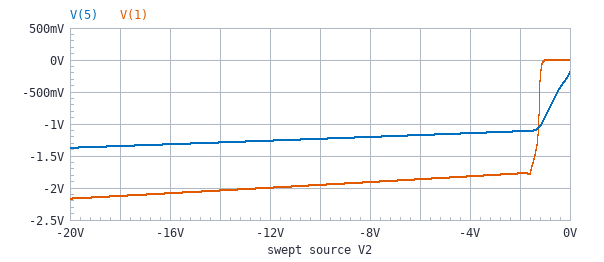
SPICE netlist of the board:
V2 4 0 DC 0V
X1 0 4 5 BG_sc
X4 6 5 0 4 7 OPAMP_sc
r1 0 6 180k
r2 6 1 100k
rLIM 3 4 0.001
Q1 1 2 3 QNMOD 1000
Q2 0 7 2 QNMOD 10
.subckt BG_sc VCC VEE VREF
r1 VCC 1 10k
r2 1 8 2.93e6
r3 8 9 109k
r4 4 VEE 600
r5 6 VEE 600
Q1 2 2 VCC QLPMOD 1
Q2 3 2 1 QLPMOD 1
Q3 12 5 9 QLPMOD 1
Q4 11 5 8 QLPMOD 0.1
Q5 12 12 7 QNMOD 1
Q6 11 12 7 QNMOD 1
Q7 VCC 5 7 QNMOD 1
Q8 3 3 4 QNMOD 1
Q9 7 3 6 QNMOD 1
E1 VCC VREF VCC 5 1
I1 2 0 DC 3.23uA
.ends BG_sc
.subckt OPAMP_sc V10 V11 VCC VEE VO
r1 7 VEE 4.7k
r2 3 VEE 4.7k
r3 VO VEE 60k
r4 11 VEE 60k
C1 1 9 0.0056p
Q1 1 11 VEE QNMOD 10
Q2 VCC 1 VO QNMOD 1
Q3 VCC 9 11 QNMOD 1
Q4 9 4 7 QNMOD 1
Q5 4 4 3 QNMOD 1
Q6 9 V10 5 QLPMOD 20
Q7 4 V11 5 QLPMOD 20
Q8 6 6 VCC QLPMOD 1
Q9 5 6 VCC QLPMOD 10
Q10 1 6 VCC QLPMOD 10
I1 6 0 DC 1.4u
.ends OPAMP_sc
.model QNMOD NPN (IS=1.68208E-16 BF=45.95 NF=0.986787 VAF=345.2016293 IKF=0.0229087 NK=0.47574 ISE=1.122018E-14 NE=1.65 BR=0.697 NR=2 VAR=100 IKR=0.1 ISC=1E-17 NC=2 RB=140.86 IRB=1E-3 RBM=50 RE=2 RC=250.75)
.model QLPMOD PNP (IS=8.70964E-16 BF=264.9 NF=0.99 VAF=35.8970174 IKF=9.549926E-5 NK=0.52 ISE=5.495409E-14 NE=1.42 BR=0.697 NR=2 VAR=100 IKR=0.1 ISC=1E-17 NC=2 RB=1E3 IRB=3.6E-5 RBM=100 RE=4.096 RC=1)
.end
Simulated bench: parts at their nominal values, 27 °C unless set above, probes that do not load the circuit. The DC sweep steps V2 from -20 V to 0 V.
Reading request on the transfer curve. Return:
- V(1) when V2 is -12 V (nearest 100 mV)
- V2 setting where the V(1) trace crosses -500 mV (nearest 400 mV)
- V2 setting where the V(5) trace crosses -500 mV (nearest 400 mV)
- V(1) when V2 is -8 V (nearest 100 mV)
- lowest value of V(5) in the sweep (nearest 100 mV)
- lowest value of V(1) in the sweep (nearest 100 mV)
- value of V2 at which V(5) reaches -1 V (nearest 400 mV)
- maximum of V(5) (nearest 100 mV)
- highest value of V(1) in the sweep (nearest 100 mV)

-2.0 V
-1.2 V
-400 mV
-1.9 V
-1.4 V
-2.2 V
-1.2 V
-200 mV
0 V
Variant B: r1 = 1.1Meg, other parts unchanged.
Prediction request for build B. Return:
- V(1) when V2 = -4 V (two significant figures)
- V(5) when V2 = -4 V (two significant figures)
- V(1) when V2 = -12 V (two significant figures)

-1.3 V
-1.1 V
-1.4 V
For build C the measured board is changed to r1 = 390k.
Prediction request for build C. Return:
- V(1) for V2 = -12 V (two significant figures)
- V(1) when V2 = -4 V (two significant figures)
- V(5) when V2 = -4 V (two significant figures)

-1.6 V
-1.5 V
-1.1 V
